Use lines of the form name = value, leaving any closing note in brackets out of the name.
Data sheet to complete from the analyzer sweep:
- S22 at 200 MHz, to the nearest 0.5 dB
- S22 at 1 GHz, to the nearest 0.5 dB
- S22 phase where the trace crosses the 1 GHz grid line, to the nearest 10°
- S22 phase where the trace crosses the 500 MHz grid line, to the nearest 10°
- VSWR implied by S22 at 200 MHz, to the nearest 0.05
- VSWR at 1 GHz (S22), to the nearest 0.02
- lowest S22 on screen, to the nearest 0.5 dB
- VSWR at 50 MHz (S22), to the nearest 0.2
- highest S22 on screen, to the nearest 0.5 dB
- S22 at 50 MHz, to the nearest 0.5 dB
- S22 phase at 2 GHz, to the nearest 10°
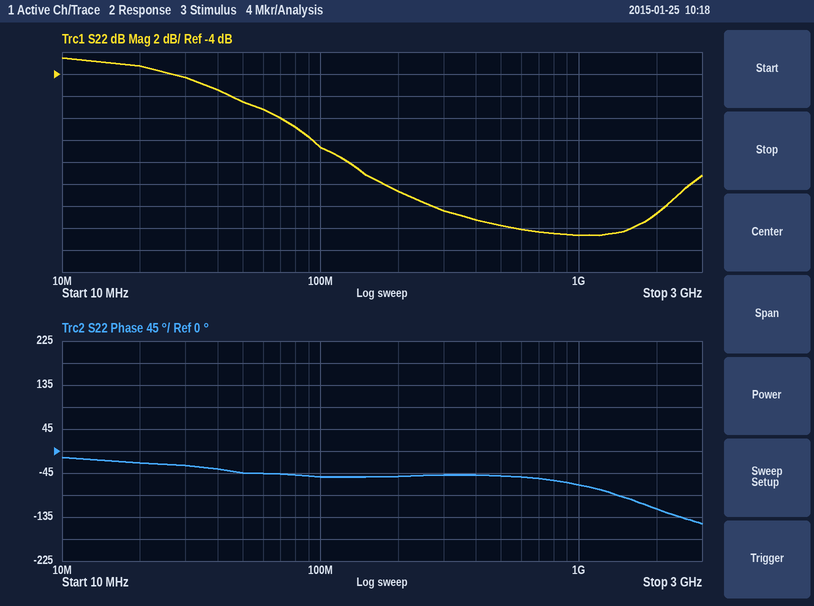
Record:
S22 at 200 MHz, to the nearest 0.5 dB = -14.5 dB
S22 at 1 GHz, to the nearest 0.5 dB = -18.5 dB
S22 phase where the trace crosses the 1 GHz grid line, to the nearest 10° = -70°
S22 phase where the trace crosses the 500 MHz grid line, to the nearest 10° = -50°
VSWR implied by S22 at 200 MHz, to the nearest 0.05 = 1.45
VSWR at 1 GHz (S22), to the nearest 0.02 = 1.26
lowest S22 on screen, to the nearest 0.5 dB = -18.5 dB
VSWR at 50 MHz (S22), to the nearest 0.2 = 2.8
highest S22 on screen, to the nearest 0.5 dB = -2.5 dB
S22 at 50 MHz, to the nearest 0.5 dB = -6.5 dB
S22 phase at 2 GHz, to the nearest 10° = -120°
